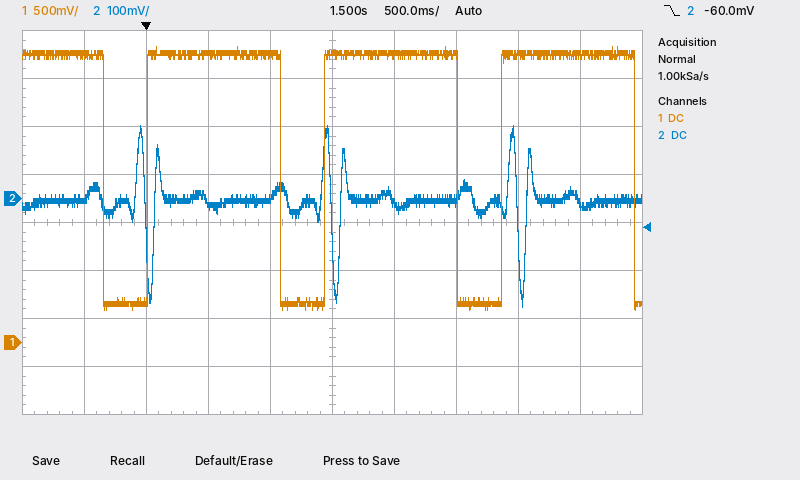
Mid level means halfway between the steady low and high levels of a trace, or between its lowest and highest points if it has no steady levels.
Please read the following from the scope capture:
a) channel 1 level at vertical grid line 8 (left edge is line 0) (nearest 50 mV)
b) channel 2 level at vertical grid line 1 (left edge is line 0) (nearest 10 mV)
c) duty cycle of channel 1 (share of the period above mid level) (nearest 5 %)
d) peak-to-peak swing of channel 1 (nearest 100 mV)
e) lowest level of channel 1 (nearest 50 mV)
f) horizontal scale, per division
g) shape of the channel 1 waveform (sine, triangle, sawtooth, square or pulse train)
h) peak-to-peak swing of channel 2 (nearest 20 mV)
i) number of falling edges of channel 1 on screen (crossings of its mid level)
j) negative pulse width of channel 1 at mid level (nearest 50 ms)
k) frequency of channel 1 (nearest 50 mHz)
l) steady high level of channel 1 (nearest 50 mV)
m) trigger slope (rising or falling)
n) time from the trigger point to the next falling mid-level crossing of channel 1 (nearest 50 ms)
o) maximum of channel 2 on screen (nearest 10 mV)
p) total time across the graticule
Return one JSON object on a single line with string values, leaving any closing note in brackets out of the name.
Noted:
{"channel 1 level at vertical grid line 8 (left edge is line 0)": "3.00 V", "channel 2 level at vertical grid line 1 (left edge is line 0)": "0 mV", "duty cycle of channel 1 (share of the period above mid level)": "75 %", "peak-to-peak swing of channel 1": "2.70 V", "lowest level of channel 1": "350 mV", "horizontal scale, per division": "500 ms", "shape of the channel 1 waveform": "pulse train", "peak-to-peak swing of channel 2": "380 mV", "number of falling edges of channel 1 on screen": "4", "negative pulse width of channel 1 at mid level": "350 ms", "frequency of channel 1": "700 mHz", "steady high level of channel 1": "3.00 V", "trigger slope": "falling", "time from the trigger point to the next falling mid-level crossing of channel 1": "1.10 s", "maximum of channel 2 on screen": "150 mV", "total time across the graticule": "5 s"}
